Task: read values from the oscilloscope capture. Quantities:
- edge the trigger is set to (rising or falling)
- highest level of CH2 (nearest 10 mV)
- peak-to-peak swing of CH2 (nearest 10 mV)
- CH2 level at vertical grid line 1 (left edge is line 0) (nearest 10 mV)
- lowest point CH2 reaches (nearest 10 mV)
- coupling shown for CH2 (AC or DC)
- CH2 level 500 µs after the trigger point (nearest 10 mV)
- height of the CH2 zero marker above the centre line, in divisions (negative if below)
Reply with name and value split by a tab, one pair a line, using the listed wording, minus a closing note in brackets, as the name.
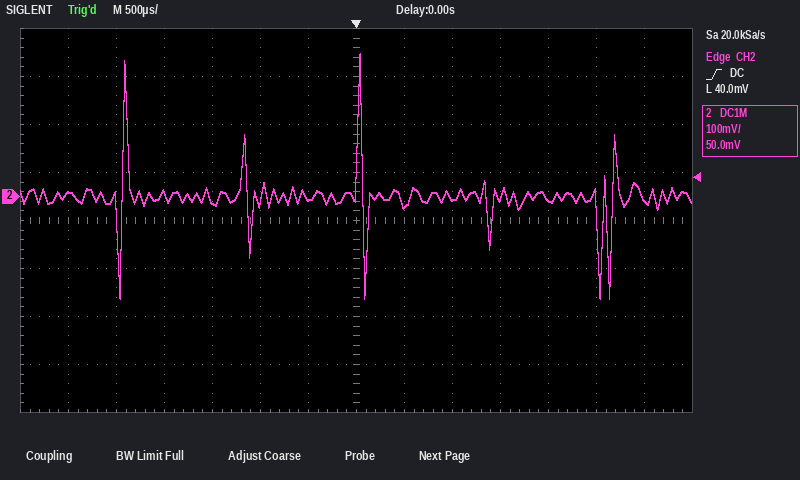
edge the trigger is set to	rising
highest level of CH2	300 mV
peak-to-peak swing of CH2	510 mV
CH2 level at vertical grid line 1 (left edge is line 0)	10 mV
lowest point CH2 reaches	-210 mV
coupling shown for CH2	DC
CH2 level 500 µs after the trigger point	-20 mV
height of the CH2 zero marker above the centre line, in divisions	+0.5 div
